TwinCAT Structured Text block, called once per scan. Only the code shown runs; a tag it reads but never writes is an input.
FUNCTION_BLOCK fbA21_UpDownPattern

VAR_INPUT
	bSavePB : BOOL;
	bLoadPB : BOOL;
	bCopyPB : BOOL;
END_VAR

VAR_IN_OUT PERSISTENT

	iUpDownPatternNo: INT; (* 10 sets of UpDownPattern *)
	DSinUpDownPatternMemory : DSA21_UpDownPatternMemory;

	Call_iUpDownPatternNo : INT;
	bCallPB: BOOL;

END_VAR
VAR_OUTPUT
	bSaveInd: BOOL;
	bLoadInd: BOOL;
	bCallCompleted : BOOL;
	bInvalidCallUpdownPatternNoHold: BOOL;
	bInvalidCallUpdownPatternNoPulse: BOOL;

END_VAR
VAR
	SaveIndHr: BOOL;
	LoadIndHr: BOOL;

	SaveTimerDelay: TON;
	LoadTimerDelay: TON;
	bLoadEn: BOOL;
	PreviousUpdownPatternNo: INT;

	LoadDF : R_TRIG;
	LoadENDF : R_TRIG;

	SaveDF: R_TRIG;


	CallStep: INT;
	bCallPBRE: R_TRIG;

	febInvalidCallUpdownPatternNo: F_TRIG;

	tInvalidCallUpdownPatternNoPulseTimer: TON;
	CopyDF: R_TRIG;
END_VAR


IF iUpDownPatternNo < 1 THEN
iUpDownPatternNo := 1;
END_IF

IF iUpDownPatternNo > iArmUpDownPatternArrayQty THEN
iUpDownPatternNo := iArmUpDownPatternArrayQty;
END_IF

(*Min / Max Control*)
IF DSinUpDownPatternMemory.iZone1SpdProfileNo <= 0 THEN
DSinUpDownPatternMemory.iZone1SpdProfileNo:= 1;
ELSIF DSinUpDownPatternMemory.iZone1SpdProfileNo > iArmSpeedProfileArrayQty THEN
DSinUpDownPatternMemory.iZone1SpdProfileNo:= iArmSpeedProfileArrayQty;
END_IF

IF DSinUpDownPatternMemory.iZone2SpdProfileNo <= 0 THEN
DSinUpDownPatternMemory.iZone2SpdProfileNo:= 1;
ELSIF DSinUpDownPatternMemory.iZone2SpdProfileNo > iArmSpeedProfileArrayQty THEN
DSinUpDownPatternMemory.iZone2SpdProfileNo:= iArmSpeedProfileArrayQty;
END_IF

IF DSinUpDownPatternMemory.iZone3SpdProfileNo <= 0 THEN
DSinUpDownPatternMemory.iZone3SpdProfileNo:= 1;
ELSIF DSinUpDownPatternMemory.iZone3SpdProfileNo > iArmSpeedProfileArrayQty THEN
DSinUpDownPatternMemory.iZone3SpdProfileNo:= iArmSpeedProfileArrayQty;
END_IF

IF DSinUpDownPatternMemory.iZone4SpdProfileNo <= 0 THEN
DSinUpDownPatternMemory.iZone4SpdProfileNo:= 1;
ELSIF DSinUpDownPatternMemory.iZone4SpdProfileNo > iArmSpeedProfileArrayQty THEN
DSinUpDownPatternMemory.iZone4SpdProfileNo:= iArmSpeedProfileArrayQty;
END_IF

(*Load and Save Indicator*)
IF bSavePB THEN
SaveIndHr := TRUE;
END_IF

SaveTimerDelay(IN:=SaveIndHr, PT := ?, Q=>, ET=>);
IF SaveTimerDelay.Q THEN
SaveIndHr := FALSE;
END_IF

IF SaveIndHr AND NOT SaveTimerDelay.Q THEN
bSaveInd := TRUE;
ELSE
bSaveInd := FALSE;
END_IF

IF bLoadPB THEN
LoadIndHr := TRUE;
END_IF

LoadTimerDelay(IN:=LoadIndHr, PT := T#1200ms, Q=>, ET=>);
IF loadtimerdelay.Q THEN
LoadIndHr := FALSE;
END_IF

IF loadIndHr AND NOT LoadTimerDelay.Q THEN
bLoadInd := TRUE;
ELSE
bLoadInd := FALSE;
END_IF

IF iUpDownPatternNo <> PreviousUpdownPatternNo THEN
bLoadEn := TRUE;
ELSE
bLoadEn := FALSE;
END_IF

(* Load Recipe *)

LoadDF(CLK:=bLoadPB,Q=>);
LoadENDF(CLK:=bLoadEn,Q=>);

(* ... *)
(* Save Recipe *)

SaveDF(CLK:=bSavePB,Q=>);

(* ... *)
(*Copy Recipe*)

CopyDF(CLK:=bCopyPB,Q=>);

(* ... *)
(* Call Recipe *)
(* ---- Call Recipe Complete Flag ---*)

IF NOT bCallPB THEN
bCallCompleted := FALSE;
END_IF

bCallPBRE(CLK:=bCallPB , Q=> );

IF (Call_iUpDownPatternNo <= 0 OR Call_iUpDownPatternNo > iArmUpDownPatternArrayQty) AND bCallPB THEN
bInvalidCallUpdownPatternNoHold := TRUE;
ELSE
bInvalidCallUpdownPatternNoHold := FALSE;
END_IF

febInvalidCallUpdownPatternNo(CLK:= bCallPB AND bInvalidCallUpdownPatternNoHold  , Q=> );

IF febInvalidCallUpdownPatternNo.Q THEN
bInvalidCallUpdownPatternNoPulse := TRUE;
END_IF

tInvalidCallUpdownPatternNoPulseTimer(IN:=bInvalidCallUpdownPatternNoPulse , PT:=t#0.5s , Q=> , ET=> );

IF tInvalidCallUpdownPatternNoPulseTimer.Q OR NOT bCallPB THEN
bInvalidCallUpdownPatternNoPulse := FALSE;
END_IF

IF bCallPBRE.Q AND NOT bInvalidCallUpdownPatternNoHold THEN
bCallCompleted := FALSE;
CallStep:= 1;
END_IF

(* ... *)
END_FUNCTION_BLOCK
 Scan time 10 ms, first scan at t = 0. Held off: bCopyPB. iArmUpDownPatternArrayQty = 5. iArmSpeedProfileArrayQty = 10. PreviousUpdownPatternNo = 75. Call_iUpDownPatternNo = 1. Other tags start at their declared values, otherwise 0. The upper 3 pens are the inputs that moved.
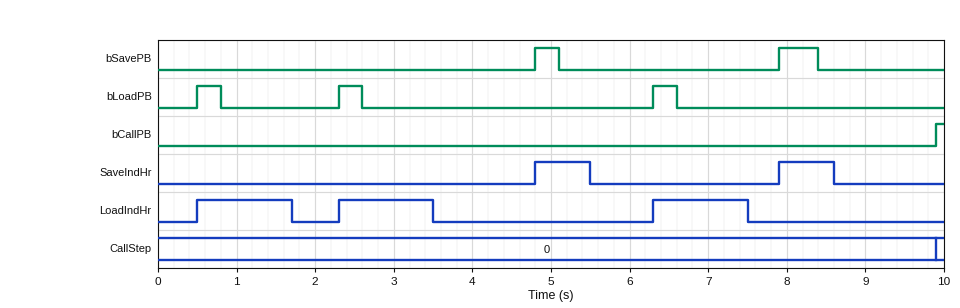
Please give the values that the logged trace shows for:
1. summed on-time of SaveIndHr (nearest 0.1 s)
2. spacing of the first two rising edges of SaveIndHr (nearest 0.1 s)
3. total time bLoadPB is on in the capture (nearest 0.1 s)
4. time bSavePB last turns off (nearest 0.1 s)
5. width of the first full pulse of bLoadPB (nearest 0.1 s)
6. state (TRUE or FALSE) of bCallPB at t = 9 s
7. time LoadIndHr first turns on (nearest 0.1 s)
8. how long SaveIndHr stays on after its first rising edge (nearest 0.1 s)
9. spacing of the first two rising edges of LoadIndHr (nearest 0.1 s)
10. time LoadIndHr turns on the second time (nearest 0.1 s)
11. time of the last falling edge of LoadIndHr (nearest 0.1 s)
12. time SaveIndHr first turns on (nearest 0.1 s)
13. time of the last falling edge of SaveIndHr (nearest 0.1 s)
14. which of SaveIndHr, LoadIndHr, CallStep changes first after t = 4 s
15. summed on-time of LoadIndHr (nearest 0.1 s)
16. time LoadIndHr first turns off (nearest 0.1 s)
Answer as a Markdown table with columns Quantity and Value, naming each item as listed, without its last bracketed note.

| Quantity | Value |
|---|---|
| summed on-time of SaveIndHr | 1.4 s |
| spacing of the first two rising edges of SaveIndHr | 3.1 s |
| total time bLoadPB is on in the capture | 0.9 s |
| time bSavePB last turns off | 8.4 s |
| width of the first full pulse of bLoadPB | 0.3 s |
| state (TRUE or FALSE) of bCallPB at t = 9 s | FALSE |
| time LoadIndHr first turns on | 0.5 s |
| how long SaveIndHr stays on after its first rising edge | 0.7 s |
| spacing of the first two rising edges of LoadIndHr | 1.8 s |
| time LoadIndHr turns on the second time | 2.3 s |
| time of the last falling edge of LoadIndHr | 7.5 s |
| time SaveIndHr first turns on | 4.8 s |
| time of the last falling edge of SaveIndHr | 8.6 s |
| which of SaveIndHr, LoadIndHr, CallStep changes first after t = 4 s | SaveIndHr |
| summed on-time of LoadIndHr | 3.6 s |
| time LoadIndHr first turns off | 1.7 s |
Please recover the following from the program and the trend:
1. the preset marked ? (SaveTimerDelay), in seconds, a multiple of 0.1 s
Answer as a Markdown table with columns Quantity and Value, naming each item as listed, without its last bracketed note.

| Quantity | Value |
|---|---|
| the preset marked ? (SaveTimerDelay), in seconds, a multiple of 0.1 s | 0.7 s |
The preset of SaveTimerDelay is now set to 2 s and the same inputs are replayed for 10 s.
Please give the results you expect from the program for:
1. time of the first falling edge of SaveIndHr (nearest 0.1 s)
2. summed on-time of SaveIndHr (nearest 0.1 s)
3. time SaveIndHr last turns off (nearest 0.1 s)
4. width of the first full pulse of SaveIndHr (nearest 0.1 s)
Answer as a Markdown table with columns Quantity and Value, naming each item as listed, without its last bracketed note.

| Quantity | Value |
|---|---|
| time of the first falling edge of SaveIndHr | 6.8 s |
| summed on-time of SaveIndHr | 4.0 s |
| time SaveIndHr last turns off | 9.9 s |
| width of the first full pulse of SaveIndHr | 2.0 s |
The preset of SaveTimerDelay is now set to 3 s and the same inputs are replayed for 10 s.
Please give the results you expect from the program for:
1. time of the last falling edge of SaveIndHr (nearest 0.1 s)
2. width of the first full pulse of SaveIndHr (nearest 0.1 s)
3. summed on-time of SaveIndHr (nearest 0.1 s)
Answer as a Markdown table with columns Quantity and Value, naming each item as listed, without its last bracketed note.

| Quantity | Value |
|---|---|
| time of the last falling edge of SaveIndHr | 7.8 s |
| width of the first full pulse of SaveIndHr | 3.0 s |
| summed on-time of SaveIndHr | 5.1 s |
